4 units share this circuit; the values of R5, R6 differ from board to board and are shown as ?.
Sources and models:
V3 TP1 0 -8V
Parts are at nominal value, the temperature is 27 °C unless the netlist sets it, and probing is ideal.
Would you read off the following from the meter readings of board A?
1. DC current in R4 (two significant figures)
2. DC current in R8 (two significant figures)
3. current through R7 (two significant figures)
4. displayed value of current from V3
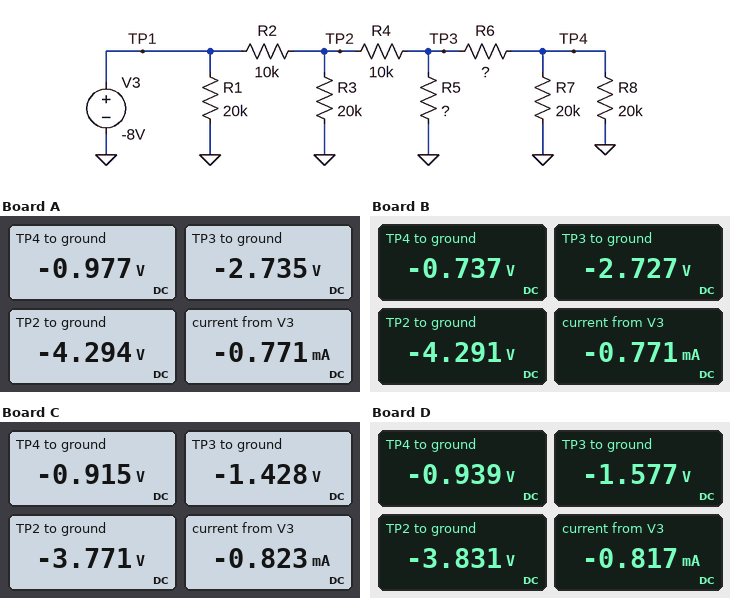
160 µA
49 µA
49 µA
-0.771 mA
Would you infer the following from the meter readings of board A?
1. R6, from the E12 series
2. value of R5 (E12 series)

18 kΩ
47 kΩ
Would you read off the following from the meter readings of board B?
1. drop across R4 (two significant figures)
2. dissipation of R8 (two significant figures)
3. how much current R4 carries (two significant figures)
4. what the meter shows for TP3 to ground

1.6 V
27 µW
160 µA
-2.727 V
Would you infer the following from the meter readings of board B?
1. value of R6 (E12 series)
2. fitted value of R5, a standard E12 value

27 kΩ
33 kΩ
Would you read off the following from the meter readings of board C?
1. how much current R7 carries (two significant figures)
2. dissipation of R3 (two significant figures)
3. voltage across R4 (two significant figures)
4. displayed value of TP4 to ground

46 µA
710 µW
2.3 V
-0.915 V
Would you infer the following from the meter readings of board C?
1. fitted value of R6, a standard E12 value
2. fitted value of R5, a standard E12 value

5.6 kΩ
10 kΩ
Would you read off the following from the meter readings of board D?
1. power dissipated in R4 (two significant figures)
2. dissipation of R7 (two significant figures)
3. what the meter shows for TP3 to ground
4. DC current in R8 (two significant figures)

510 µW
44 µW
-1.577 V
47 µA
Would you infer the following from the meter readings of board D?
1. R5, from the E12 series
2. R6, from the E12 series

12 kΩ
6.8 kΩ
